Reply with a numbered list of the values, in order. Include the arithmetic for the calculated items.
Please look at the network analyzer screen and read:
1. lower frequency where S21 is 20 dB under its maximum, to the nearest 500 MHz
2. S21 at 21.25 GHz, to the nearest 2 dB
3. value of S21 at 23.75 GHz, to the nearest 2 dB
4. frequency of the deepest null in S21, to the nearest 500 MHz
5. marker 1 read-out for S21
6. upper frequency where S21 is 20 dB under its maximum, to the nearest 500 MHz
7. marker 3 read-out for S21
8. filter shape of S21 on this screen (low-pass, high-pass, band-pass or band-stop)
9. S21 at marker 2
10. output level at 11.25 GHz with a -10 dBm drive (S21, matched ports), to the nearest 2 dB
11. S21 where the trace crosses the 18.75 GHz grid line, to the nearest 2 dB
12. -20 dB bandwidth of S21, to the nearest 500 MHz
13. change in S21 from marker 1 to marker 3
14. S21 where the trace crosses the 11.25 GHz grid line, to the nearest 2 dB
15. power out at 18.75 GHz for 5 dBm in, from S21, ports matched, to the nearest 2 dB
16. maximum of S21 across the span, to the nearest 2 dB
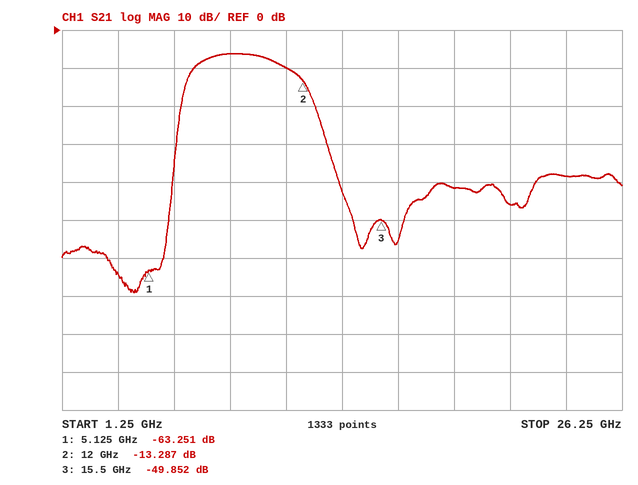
1. 6.5 GHz
2. -46 dB
3. -38 dB
4. 4.5 GHz
5. -63.251 dB
6. 13.0 GHz
7. -49.852 dB
8. band-pass
9. -13.287 dB
10. -10 dBm + (-10 dB) = -20 dBm
11. -42 dB
12. 13.0 GHz − 6.5 GHz = 6.5 GHz
13. -49.852 − (-63.251) = 13.399 dB
14. -10 dB
15. 5 dBm + (-42 dB) = -36 dBm
16. -6 dB
